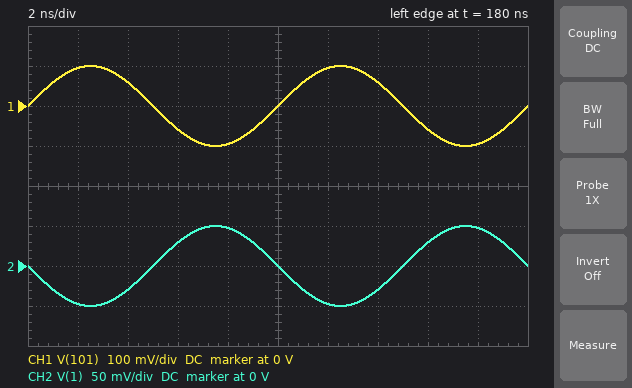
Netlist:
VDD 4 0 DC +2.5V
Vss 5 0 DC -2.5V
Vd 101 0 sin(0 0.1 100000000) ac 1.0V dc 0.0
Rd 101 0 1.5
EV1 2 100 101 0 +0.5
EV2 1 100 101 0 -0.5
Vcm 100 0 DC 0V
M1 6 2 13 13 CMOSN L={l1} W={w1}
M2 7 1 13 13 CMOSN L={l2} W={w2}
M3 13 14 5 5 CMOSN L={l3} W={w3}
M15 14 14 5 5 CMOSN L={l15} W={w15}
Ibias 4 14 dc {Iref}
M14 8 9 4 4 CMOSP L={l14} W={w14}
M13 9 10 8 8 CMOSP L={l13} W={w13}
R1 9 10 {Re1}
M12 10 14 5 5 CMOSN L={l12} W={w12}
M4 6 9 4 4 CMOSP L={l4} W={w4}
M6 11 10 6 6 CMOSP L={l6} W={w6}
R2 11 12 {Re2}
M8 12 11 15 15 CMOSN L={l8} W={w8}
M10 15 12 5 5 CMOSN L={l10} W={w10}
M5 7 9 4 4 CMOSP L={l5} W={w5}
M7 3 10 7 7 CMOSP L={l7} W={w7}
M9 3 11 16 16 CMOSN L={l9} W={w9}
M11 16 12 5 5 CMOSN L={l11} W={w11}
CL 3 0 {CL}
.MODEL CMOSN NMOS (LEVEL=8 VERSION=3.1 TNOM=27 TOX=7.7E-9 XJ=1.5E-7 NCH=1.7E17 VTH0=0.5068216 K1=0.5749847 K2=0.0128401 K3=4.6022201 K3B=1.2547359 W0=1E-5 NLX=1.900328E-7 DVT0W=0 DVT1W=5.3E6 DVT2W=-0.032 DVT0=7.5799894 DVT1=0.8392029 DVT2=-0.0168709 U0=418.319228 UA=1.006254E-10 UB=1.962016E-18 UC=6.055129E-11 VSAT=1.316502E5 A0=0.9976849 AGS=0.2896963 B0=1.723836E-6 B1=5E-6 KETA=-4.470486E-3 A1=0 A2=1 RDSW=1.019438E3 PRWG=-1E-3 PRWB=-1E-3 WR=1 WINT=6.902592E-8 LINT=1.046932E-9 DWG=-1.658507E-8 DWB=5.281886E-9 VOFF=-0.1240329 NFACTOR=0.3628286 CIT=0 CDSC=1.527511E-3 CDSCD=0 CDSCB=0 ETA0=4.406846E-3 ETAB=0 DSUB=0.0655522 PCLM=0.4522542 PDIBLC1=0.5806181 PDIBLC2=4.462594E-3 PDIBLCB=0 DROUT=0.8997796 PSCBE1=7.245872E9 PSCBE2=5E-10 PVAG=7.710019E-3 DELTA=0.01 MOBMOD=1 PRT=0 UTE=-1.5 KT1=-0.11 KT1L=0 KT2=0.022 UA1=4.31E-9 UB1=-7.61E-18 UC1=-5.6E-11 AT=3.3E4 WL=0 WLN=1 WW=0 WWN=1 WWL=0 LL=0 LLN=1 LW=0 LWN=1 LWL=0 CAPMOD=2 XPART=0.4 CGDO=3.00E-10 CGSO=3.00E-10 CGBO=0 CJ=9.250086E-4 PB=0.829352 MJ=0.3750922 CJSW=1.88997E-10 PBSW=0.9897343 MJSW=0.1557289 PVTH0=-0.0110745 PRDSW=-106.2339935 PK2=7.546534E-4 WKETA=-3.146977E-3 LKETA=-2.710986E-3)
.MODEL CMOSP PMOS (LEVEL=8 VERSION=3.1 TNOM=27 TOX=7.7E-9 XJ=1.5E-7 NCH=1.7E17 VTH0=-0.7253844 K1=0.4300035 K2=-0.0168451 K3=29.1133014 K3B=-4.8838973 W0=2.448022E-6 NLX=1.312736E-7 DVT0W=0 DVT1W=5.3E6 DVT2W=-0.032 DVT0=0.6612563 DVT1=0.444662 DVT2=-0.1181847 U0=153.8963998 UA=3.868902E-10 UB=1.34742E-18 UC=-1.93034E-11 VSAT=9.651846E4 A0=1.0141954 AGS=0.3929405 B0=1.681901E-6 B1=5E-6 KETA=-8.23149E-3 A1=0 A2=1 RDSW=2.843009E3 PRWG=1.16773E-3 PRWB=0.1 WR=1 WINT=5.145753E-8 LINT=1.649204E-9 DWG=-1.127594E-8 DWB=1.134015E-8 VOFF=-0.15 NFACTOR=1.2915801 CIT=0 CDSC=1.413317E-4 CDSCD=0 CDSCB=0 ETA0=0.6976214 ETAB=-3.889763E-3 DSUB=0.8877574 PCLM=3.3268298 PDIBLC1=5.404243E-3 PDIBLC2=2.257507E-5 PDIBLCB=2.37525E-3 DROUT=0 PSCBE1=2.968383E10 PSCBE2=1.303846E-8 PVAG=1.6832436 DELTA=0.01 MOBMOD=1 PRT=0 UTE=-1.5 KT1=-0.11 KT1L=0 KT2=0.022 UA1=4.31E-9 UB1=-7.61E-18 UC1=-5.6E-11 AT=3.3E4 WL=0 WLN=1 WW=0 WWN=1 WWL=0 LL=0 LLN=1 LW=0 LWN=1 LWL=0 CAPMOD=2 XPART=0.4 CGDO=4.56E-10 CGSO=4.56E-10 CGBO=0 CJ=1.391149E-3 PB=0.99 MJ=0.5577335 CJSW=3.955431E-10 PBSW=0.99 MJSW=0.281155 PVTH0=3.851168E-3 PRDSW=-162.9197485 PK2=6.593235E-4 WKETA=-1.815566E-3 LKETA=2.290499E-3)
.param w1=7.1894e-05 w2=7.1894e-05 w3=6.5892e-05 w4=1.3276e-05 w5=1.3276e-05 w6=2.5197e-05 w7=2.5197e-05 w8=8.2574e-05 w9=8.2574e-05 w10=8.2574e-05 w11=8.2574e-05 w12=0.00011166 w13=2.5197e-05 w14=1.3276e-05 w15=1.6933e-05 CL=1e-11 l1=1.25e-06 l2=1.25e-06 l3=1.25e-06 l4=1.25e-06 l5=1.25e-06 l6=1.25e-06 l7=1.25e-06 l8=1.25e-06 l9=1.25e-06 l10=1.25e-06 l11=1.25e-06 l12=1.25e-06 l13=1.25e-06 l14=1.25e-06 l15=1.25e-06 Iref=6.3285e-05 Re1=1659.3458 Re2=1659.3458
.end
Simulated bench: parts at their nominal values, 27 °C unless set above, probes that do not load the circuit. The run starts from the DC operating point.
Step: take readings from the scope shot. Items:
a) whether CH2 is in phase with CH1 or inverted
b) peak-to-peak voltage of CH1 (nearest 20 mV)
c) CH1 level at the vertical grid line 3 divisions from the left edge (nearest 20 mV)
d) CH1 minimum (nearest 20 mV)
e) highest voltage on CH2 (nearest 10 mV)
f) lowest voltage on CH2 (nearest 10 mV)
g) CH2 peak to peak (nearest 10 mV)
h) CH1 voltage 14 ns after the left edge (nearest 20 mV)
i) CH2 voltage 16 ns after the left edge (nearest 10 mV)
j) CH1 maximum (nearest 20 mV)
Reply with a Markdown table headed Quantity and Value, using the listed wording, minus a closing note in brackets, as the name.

| Quantity | Value |
|---|---|
| whether CH2 is in phase with CH1 or inverted | inverted |
| peak-to-peak voltage of CH1 | 200 mV |
| CH1 level at the vertical grid line 3 divisions from the left edge | -60 mV |
| CH1 minimum | -100 mV |
| highest voltage on CH2 | 50 mV |
| lowest voltage on CH2 | -50 mV |
| CH2 peak to peak | 100 mV |
| CH1 voltage 14 ns after the left edge | 60 mV |
| CH2 voltage 16 ns after the left edge | 30 mV |
| CH1 maximum | 100 mV |
